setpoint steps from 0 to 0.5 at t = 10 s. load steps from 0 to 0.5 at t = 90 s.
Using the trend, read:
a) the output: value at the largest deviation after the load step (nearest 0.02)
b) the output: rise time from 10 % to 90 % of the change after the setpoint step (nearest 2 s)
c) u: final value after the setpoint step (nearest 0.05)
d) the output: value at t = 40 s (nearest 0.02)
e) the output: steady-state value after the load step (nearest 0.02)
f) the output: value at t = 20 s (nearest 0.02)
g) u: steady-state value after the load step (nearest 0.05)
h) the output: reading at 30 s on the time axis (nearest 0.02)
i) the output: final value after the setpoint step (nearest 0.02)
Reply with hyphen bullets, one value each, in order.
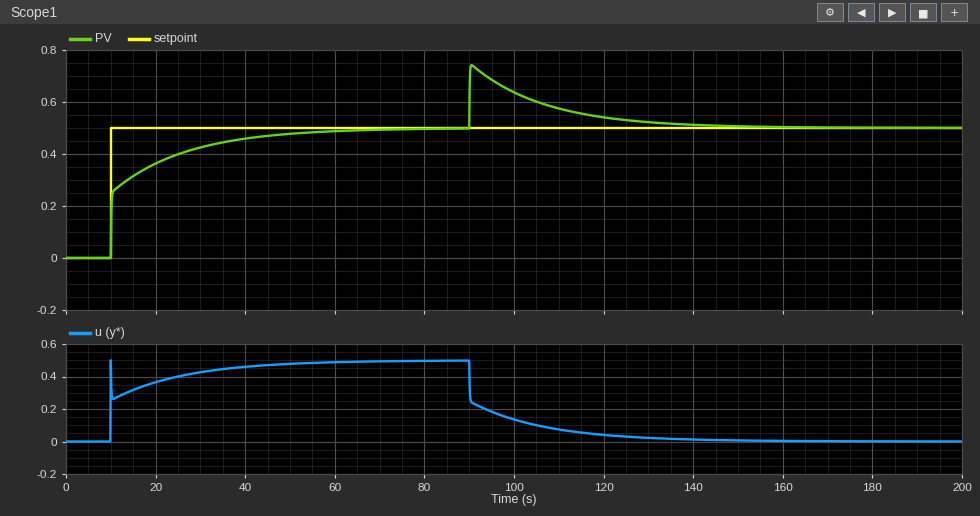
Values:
- 0.74
- 26 s
- 0.50
- 0.46
- 0.50
- 0.36
- 0.00
- 0.42
- 0.50
